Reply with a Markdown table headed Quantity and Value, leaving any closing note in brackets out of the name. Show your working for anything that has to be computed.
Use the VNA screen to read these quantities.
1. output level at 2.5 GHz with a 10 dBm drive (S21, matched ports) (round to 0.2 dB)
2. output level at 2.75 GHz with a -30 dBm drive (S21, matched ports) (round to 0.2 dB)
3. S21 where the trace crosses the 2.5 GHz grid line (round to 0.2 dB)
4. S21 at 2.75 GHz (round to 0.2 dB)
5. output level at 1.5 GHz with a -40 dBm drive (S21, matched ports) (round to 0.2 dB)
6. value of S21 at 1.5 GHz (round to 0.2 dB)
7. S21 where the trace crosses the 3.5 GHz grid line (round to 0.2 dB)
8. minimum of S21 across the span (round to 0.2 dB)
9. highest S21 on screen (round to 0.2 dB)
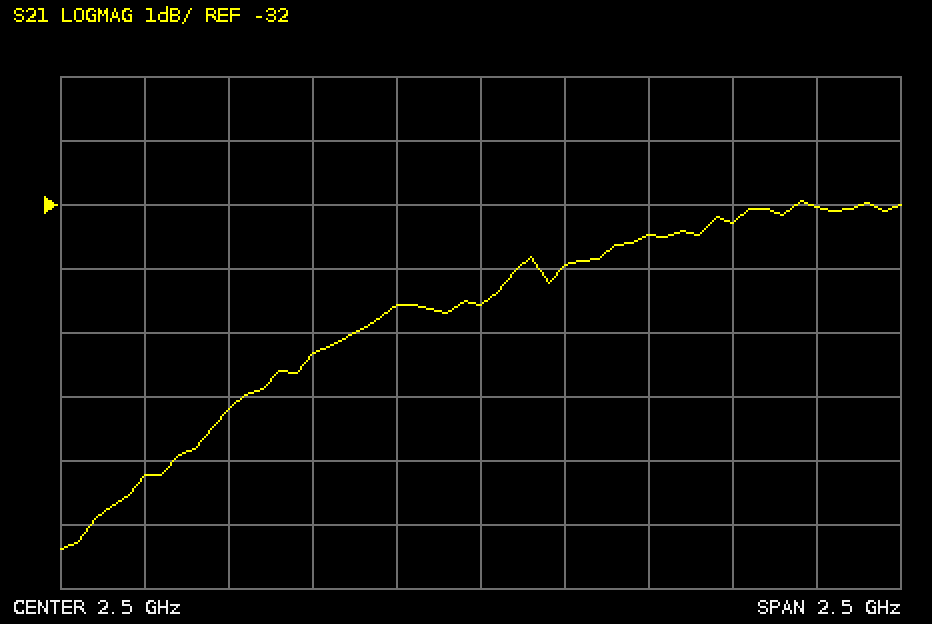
| Quantity | Value |
|---|---|
| output level at 2.5 GHz with a 10 dBm drive (S21, matched ports) | 10 dBm + (-33.6 dB) = -23.6 dBm |
| output level at 2.75 GHz with a -30 dBm drive (S21, matched ports) | -30 dBm + (-33.0 dB) = -63.0 dBm |
| S21 where the trace crosses the 2.5 GHz grid line | -33.6 dB |
| S21 at 2.75 GHz | -33.0 dB |
| output level at 1.5 GHz with a -40 dBm drive (S21, matched ports) | -40 dBm + (-36.2 dB) = -76.2 dBm |
| value of S21 at 1.5 GHz | -36.2 dB |
| S21 where the trace crosses the 3.5 GHz grid line | -32.0 dB |
| minimum of S21 across the span | -37.4 dB |
| highest S21 on screen | -32.0 dB |
